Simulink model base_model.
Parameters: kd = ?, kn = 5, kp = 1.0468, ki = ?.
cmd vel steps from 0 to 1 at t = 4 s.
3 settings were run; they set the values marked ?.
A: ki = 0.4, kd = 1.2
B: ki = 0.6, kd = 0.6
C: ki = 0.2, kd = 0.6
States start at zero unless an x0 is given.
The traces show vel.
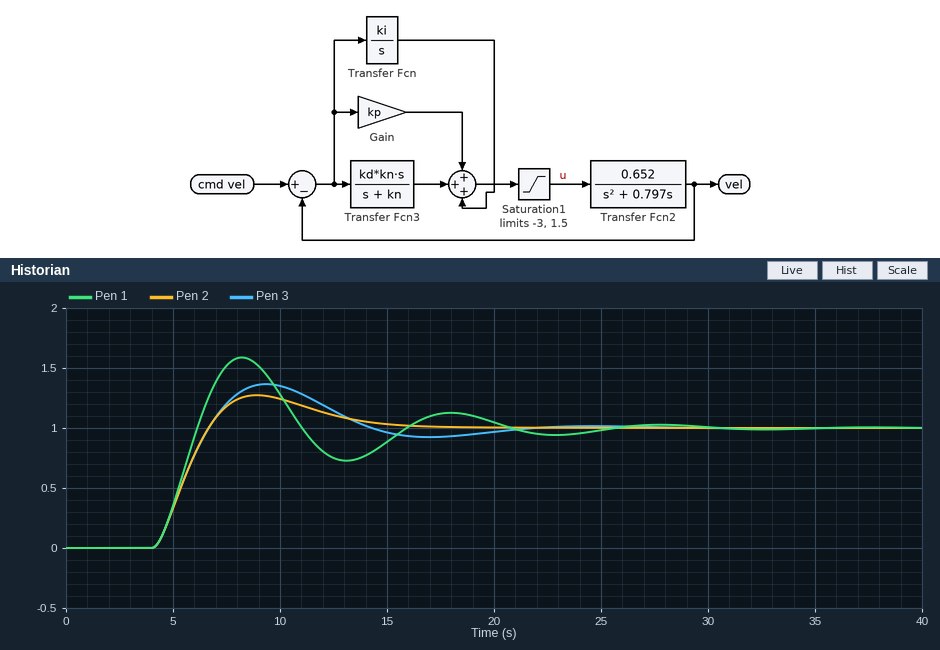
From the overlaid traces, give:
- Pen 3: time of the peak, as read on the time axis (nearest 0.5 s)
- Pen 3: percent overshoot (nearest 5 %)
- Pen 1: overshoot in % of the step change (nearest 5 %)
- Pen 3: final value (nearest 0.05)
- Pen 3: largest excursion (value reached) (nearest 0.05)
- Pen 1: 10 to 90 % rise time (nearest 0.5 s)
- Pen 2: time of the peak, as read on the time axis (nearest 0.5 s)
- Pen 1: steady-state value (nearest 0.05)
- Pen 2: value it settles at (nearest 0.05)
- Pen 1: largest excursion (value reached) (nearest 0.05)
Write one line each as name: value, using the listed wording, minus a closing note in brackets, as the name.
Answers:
Pen 3: time of the peak, as read on the time axis: 9.5 s
Pen 3: percent overshoot: 35 %
Pen 1: overshoot in % of the step change: 60 %
Pen 3: final value: 1.00
Pen 3: largest excursion (value reached): 1.35
Pen 1: 10 to 90 % rise time: 1.5 s
Pen 2: time of the peak, as read on the time axis: 9.0 s
Pen 1: steady-state value: 1.00
Pen 2: value it settles at: 1.00
Pen 1: largest excursion (value reached): 1.60
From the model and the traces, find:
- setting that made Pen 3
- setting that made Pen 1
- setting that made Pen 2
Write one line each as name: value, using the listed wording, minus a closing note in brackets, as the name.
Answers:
setting that made Pen 3: A
setting that made Pen 1: B
setting that made Pen 2: C
